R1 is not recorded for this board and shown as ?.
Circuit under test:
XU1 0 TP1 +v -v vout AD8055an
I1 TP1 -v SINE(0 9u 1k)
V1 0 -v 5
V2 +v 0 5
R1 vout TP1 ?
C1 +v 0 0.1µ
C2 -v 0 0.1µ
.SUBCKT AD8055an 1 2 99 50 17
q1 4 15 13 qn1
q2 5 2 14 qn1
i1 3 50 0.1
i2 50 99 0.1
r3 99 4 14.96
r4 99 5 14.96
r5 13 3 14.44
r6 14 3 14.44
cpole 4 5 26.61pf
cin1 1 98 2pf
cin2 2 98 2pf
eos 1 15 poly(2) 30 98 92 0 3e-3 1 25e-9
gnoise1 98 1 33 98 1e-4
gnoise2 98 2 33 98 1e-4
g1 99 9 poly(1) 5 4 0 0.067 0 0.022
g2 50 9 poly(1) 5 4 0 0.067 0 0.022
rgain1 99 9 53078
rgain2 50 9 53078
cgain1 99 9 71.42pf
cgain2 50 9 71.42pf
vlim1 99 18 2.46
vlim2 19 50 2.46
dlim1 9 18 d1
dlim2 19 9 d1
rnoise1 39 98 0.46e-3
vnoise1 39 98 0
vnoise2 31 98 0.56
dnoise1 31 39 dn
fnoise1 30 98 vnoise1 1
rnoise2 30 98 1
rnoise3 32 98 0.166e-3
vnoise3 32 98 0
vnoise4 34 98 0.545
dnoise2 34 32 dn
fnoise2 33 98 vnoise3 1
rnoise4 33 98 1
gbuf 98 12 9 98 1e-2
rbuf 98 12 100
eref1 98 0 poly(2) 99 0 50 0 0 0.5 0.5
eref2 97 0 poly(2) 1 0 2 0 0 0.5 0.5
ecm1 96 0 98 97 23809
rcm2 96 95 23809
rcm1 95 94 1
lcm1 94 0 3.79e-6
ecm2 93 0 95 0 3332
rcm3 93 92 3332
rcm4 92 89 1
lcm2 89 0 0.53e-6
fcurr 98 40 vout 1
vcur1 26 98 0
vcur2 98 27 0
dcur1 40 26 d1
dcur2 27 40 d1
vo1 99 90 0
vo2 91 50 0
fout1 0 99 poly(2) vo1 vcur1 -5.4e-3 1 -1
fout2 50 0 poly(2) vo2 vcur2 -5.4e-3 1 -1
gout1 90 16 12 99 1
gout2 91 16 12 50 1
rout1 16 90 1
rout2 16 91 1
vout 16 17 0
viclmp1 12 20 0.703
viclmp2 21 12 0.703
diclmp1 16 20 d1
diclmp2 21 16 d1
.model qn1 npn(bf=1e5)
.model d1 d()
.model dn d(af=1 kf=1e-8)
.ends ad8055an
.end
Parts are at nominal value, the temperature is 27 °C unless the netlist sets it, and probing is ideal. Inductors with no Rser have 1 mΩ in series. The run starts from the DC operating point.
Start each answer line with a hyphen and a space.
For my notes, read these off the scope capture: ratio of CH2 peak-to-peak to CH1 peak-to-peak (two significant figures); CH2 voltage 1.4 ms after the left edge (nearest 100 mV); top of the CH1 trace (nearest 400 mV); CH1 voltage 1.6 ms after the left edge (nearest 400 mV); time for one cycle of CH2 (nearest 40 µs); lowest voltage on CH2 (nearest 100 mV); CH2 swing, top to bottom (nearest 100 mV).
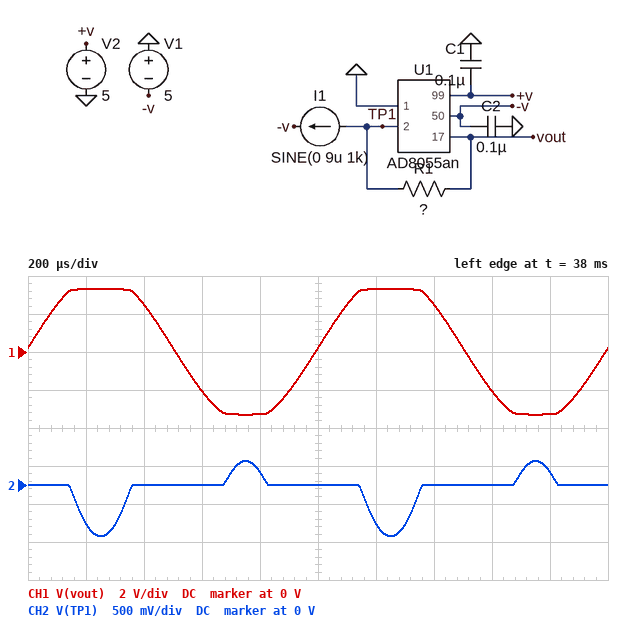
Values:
- 0.15
- 0 V
- 3.2 V
- -2.0 V
- 1.00 ms
- -700 mV
- 1.0 V
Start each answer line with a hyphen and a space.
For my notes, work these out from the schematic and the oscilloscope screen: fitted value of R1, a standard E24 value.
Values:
- 430 kΩ
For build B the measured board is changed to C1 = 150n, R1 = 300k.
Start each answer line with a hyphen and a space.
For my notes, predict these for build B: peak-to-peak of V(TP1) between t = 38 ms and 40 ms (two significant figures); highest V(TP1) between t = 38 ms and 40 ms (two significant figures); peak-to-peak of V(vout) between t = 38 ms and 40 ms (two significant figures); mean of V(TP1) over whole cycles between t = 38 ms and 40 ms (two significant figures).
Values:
- 1.5 mV
- -2.3 mV
- 5.4 V
- -3.0 mV
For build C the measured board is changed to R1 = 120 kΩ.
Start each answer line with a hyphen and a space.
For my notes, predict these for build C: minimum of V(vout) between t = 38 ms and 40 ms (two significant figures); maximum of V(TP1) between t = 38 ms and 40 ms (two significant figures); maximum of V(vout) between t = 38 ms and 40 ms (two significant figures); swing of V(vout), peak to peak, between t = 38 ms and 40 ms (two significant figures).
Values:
- -1.0 V
- -2.7 mV
- 1.1 V
- 2.2 V
